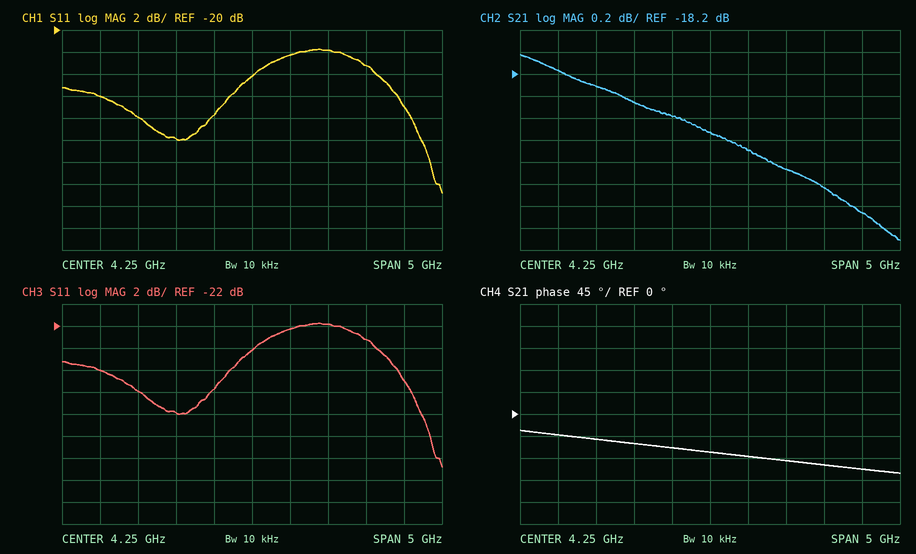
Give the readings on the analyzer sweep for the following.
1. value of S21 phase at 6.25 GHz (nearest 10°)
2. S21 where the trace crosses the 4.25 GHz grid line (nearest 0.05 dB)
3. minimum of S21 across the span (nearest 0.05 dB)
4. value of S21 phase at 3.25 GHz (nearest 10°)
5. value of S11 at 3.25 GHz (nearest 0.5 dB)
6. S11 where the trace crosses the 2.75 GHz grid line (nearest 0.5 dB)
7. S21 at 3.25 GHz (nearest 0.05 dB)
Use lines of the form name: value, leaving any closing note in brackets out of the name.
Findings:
value of S21 phase at 6.25 GHz: -110°
S21 where the trace crosses the 4.25 GHz grid line: -18.75 dB
minimum of S21 across the span: -19.70 dB
value of S21 phase at 3.25 GHz: -60°
value of S11 at 3.25 GHz: -30.0 dB
S11 where the trace crosses the 2.75 GHz grid line: -28.0 dB
S21 at 3.25 GHz: -18.45 dB
